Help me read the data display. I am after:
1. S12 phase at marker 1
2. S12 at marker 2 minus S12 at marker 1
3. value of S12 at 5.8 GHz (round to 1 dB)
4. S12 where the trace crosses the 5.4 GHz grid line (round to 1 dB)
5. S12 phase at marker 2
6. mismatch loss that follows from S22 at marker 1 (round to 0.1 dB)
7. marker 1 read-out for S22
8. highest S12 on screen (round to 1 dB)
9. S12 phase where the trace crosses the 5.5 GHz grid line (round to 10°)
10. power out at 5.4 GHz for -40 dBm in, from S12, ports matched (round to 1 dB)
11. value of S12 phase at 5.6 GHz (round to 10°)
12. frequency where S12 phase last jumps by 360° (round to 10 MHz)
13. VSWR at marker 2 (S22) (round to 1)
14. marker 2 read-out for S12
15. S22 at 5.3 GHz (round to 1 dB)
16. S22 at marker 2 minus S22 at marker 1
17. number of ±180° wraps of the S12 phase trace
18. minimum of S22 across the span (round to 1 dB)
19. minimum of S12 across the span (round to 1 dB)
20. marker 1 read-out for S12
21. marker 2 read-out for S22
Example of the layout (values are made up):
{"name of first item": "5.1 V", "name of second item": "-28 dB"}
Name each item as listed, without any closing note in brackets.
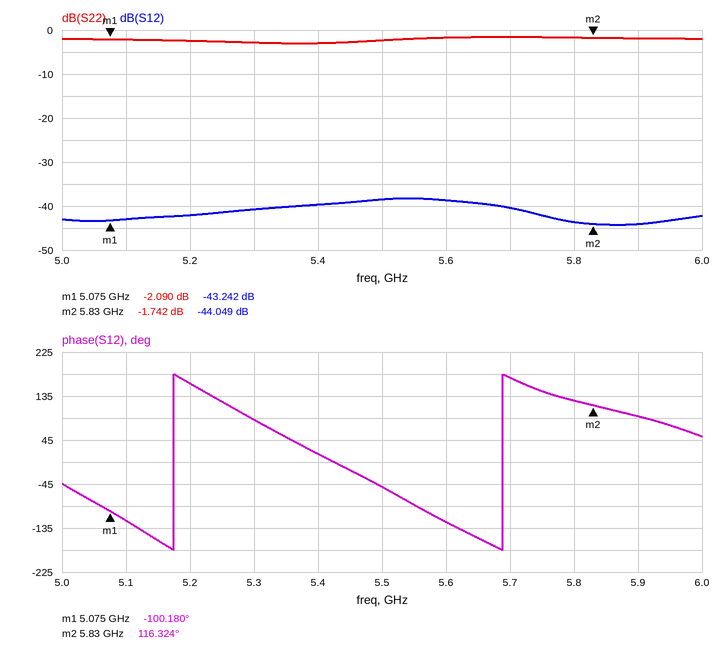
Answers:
{"S12 phase at marker 1": "-100.180°", "S12 at marker 2 minus S12 at marker 1": "-0.807 dB", "value of S12 at 5.8 GHz": "-44 dB", "S12 where the trace crosses the 5.4 GHz grid line": "-40 dB", "S12 phase at marker 2": "116.324°", "mismatch loss that follows from S22 at marker 1": "4.2 dB", "marker 1 read-out for S22": "-2.090 dB", "highest S12 on screen": "-38 dB", "S12 phase where the trace crosses the 5.5 GHz grid line": "-50°", "power out at 5.4 GHz for -40 dBm in, from S12, ports matched": "-80 dBm", "value of S12 phase at 5.6 GHz": "-120°", "frequency where S12 phase last jumps by 360°": "5.69 GHz", "VSWR at marker 2 (S22)": "10", "marker 2 read-out for S12": "-44.049 dB", "S22 at 5.3 GHz": "-3 dB", "S22 at marker 2 minus S22 at marker 1": "0.348 dB", "number of ±180° wraps of the S12 phase trace": "2", "minimum of S22 across the span": "-3 dB", "minimum of S12 across the span": "-44 dB", "marker 1 read-out for S12": "-43.242 dB", "marker 2 read-out for S22": "-1.742 dB"}
